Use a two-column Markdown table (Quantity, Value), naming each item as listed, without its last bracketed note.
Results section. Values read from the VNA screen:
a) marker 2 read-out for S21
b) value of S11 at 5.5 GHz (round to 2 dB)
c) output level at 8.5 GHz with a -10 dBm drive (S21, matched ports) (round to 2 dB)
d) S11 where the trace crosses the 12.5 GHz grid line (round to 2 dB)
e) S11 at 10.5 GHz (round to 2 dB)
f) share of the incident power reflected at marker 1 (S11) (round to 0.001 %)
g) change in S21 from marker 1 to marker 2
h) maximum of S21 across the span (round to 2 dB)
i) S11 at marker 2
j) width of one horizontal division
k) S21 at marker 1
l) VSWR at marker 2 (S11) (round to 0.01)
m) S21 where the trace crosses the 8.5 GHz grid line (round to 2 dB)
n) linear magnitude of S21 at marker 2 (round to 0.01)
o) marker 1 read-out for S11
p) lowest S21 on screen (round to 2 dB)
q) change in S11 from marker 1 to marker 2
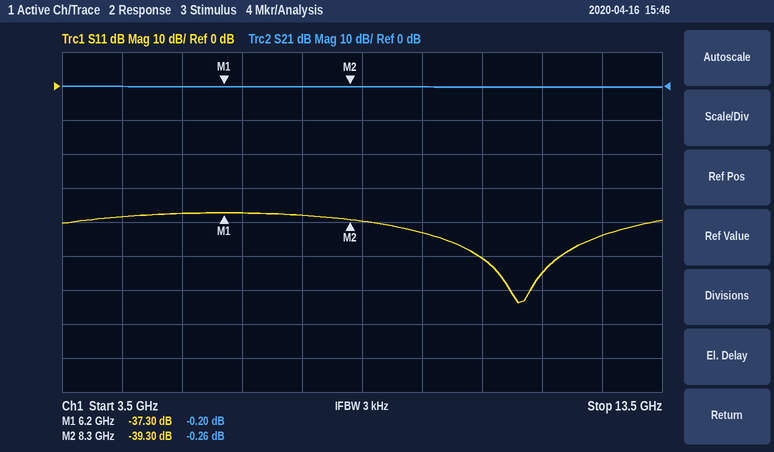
| Quantity | Value |
|---|---|
| marker 2 read-out for S21 | -0.26 dB |
| value of S11 at 5.5 GHz | -38 dB |
| output level at 8.5 GHz with a -10 dBm drive (S21, matched ports) | -10 dBm |
| S11 where the trace crosses the 12.5 GHz grid line | -44 dB |
| S11 at 10.5 GHz | -50 dB |
| share of the incident power reflected at marker 1 (S11) | 0.019 % |
| change in S21 from marker 1 to marker 2 | -0.06 dB |
| maximum of S21 across the span | 0 dB |
| S11 at marker 2 | -39.30 dB |
| width of one horizontal division | 1 GHz |
| S21 at marker 1 | -0.20 dB |
| VSWR at marker 2 (S11) | 1.02 |
| S21 where the trace crosses the 8.5 GHz grid line | 0 dB |
| linear magnitude of S21 at marker 2 | 0.97 |
| marker 1 read-out for S11 | -37.30 dB |
| lowest S21 on screen | 0 dB |
| change in S11 from marker 1 to marker 2 | -2.00 dB |
